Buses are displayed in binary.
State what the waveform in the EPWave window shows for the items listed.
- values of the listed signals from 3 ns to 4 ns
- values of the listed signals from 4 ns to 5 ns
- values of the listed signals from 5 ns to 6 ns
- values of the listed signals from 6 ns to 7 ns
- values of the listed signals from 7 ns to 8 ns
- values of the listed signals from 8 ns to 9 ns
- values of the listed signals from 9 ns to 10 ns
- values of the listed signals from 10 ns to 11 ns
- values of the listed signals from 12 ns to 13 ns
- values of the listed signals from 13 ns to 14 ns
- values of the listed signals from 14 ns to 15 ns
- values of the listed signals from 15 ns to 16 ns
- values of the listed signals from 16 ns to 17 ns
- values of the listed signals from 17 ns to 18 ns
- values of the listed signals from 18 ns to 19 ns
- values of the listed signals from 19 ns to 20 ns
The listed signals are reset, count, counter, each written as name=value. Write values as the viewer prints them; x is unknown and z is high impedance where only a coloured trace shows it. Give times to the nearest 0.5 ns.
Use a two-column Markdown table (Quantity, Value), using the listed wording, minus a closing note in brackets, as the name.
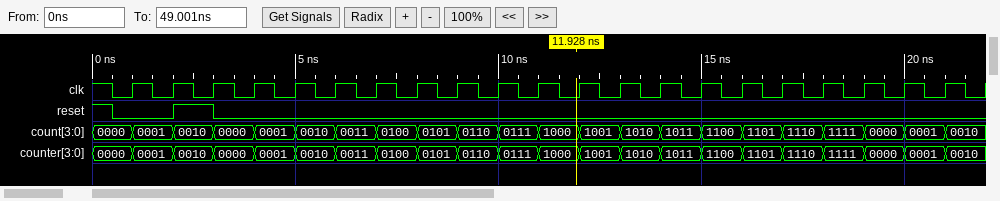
| Quantity | Value |
|---|---|
| values of the listed signals from 3 ns to 4 ns | reset=0, count=0000, counter=0000 |
| values of the listed signals from 4 ns to 5 ns | reset=0, count=0001, counter=0001 |
| values of the listed signals from 5 ns to 6 ns | reset=0, count=0010, counter=0010 |
| values of the listed signals from 6 ns to 7 ns | reset=0, count=0011, counter=0011 |
| values of the listed signals from 7 ns to 8 ns | reset=0, count=0100, counter=0100 |
| values of the listed signals from 8 ns to 9 ns | reset=0, count=0101, counter=0101 |
| values of the listed signals from 9 ns to 10 ns | reset=0, count=0110, counter=0110 |
| values of the listed signals from 10 ns to 11 ns | reset=0, count=0111, counter=0111 |
| values of the listed signals from 12 ns to 13 ns | reset=0, count=1001, counter=1001 |
| values of the listed signals from 13 ns to 14 ns | reset=0, count=1010, counter=1010 |
| values of the listed signals from 14 ns to 15 ns | reset=0, count=1011, counter=1011 |
| values of the listed signals from 15 ns to 16 ns | reset=0, count=1100, counter=1100 |
| values of the listed signals from 16 ns to 17 ns | reset=0, count=1101, counter=1101 |
| values of the listed signals from 17 ns to 18 ns | reset=0, count=1110, counter=1110 |
| values of the listed signals from 18 ns to 19 ns | reset=0, count=1111, counter=1111 |
| values of the listed signals from 19 ns to 20 ns | reset=0, count=0000, counter=0000 |
